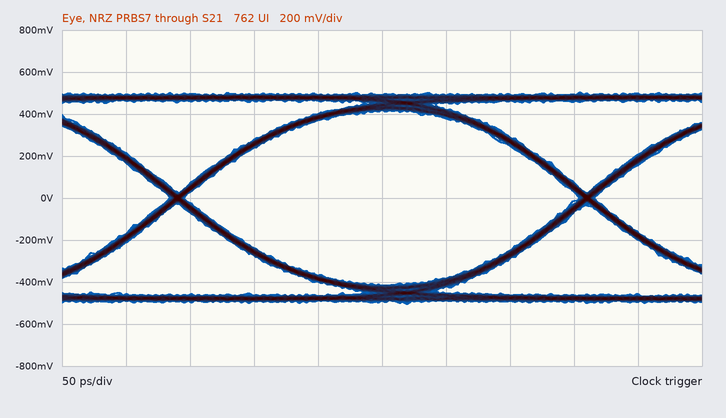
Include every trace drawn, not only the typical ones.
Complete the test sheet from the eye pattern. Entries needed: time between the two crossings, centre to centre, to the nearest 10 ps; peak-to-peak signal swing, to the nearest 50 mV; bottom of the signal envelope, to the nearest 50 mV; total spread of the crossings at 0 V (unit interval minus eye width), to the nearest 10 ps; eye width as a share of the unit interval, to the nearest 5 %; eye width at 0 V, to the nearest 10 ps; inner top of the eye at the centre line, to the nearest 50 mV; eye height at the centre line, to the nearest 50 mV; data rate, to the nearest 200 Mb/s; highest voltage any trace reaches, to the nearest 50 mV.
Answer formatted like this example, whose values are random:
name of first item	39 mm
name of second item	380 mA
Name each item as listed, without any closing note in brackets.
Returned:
time between the two crossings, centre to centre, to the nearest 10 ps	320 ps
peak-to-peak signal swing, to the nearest 50 mV	1.00 V
bottom of the signal envelope, to the nearest 50 mV	-500 mV
total spread of the crossings at 0 V (unit interval minus eye width), to the nearest 10 ps	10 ps
eye width as a share of the unit interval, to the nearest 5 %	95 %
eye width at 0 V, to the nearest 10 ps	310 ps
inner top of the eye at the centre line, to the nearest 50 mV	400 mV
eye height at the centre line, to the nearest 50 mV	850 mV
data rate, to the nearest 200 Mb/s	3.2 Gb/s
highest voltage any trace reaches, to the nearest 50 mV	500 mV
